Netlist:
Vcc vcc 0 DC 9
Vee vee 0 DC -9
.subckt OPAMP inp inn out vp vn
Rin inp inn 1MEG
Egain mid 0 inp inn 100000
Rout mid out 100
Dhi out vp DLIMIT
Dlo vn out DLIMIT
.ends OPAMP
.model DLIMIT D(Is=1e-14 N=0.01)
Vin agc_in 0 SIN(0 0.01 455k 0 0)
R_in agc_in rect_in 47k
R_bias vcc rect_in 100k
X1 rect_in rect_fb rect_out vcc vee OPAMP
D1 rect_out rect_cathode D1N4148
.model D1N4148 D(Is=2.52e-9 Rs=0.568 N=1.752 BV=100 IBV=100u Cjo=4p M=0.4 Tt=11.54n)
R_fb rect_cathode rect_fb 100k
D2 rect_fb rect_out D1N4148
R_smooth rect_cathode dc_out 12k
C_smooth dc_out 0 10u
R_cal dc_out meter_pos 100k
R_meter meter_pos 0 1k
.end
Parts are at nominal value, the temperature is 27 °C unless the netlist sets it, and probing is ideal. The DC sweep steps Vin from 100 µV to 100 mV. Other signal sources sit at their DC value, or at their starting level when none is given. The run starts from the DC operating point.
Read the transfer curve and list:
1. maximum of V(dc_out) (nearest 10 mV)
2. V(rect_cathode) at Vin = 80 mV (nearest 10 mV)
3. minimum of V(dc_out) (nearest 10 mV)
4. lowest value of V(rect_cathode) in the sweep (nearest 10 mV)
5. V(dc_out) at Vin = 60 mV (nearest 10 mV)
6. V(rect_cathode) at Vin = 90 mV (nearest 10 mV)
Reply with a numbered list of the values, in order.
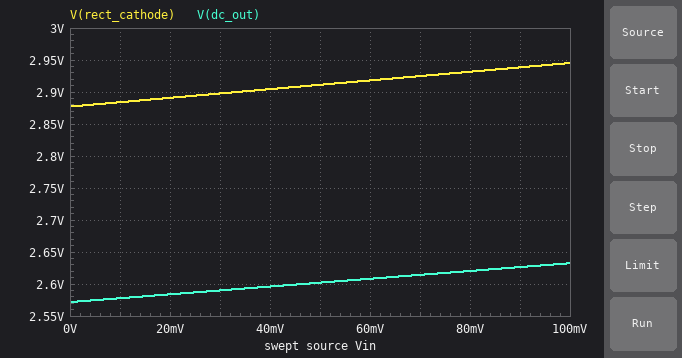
1. 2.63 V
2. 2.93 V
3. 2.57 V
4. 2.88 V
5. 2.61 V
6. 2.94 V
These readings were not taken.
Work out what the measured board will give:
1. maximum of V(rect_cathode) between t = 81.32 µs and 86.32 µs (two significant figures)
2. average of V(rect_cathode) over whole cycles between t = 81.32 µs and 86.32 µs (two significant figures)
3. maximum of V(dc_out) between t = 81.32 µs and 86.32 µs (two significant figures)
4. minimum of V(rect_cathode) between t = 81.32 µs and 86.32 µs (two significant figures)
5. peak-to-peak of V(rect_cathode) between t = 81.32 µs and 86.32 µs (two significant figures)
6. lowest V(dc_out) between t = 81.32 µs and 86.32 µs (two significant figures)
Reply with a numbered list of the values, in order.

1. 2.9 V
2. 2.9 V
3. 2.6 V
4. 2.9 V
5. 13 mV
6. 2.6 V
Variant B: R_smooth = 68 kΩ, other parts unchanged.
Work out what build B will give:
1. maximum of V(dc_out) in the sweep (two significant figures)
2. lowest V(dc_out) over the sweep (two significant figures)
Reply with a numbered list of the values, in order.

1. 1.8 V
2. 1.7 V
